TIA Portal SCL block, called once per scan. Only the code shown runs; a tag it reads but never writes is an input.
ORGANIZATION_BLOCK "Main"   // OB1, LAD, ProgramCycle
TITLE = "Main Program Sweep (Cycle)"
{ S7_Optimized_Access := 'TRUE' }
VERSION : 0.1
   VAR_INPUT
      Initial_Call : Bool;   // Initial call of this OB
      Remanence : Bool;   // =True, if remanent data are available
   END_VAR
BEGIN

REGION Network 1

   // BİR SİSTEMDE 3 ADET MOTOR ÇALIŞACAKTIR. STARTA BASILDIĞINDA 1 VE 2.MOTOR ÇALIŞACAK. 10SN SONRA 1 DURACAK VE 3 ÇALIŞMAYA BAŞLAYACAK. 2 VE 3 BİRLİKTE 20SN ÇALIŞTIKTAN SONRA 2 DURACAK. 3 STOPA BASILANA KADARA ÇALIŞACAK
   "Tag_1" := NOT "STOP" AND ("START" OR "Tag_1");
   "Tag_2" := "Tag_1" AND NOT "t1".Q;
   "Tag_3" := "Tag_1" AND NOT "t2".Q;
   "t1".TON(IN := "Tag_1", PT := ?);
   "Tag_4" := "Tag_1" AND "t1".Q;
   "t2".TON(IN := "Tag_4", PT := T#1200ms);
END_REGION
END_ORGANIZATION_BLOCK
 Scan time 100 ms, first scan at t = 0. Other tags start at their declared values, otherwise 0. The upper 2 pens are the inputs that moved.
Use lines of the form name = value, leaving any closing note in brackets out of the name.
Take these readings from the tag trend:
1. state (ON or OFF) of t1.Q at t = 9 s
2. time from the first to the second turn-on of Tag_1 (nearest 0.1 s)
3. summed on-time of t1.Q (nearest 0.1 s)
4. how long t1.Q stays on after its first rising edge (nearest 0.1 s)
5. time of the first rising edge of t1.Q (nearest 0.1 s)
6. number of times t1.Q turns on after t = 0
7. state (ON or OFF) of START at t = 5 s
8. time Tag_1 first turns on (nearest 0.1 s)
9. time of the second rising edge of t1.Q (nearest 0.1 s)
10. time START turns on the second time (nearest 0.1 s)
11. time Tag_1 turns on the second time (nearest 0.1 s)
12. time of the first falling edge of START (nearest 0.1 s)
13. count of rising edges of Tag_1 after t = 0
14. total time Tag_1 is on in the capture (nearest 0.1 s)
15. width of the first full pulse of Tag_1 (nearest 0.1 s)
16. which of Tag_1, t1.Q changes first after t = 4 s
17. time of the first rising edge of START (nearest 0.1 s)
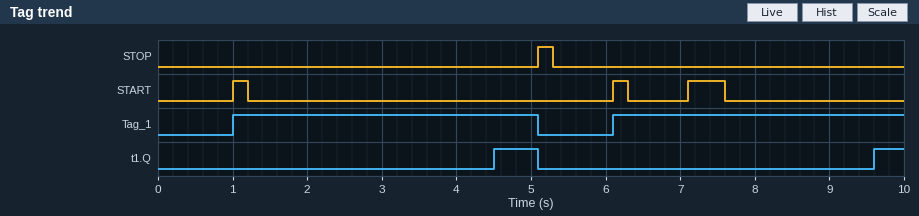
state (ON or OFF) of t1.Q at t = 9 s = OFF
time from the first to the second turn-on of Tag_1 = 5.1 s
summed on-time of t1.Q = 1.0 s
how long t1.Q stays on after its first rising edge = 0.6 s
time of the first rising edge of t1.Q = 4.5 s
number of times t1.Q turns on after t = 0 = 2
state (ON or OFF) of START at t = 5 s = OFF
time Tag_1 first turns on = 1.0 s
time of the second rising edge of t1.Q = 9.6 s
time START turns on the second time = 6.1 s
time Tag_1 turns on the second time = 6.1 s
time of the first falling edge of START = 1.2 s
count of rising edges of Tag_1 after t = 0 = 2
total time Tag_1 is on in the capture = 8.0 s
width of the first full pulse of Tag_1 = 4.1 s
which of Tag_1, t1.Q changes first after t = 4 s = t1.Q
time of the first rising edge of START = 1.0 s
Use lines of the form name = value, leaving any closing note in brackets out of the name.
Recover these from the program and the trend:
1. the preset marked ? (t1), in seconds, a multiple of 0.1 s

the preset marked ? (t1), in seconds, a multiple of 0.1 s = 3.5 s
